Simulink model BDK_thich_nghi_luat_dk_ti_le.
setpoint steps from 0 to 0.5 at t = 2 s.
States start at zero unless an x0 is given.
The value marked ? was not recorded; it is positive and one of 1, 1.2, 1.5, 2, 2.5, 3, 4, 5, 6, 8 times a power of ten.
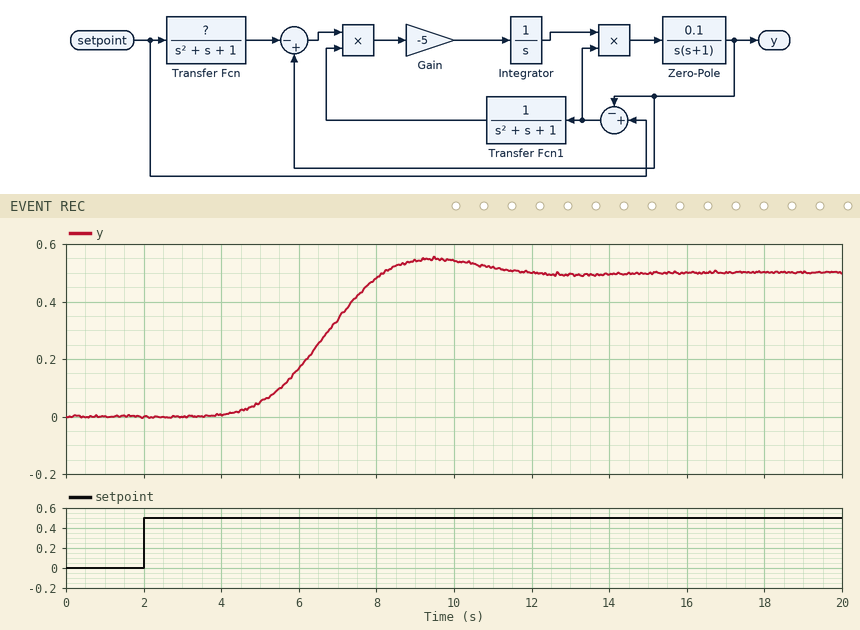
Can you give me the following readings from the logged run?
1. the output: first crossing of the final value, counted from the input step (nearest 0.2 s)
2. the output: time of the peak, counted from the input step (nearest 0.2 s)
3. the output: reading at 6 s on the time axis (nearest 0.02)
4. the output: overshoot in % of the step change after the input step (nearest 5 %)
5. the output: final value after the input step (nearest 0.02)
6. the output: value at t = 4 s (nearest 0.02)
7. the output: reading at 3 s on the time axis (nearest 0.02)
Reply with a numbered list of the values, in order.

1. 6.2 s
2. 7.4 s
3. 0.16
4. 10 %
5. 0.50
6. 0.00
7. 0.00
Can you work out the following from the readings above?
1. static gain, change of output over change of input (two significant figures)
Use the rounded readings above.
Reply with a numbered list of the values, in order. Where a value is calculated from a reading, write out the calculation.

1. (0.5 - 0) / (0.5 - 0) = 1.0
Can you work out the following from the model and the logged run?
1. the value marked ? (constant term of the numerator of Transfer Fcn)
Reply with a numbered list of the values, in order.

1. 2
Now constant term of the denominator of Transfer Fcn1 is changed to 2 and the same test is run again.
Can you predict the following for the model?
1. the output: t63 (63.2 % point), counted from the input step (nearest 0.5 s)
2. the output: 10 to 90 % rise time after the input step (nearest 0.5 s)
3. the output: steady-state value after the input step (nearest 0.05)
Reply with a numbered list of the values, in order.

1. 5.5 s
2. 4.0 s
3. 0.50
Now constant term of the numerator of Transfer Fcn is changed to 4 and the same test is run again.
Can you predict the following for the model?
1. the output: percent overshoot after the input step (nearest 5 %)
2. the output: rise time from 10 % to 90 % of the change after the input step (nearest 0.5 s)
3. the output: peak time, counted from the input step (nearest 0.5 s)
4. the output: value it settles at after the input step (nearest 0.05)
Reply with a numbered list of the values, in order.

1. 15 %
2. 2.0 s
3. 6.0 s
4. 0.50
